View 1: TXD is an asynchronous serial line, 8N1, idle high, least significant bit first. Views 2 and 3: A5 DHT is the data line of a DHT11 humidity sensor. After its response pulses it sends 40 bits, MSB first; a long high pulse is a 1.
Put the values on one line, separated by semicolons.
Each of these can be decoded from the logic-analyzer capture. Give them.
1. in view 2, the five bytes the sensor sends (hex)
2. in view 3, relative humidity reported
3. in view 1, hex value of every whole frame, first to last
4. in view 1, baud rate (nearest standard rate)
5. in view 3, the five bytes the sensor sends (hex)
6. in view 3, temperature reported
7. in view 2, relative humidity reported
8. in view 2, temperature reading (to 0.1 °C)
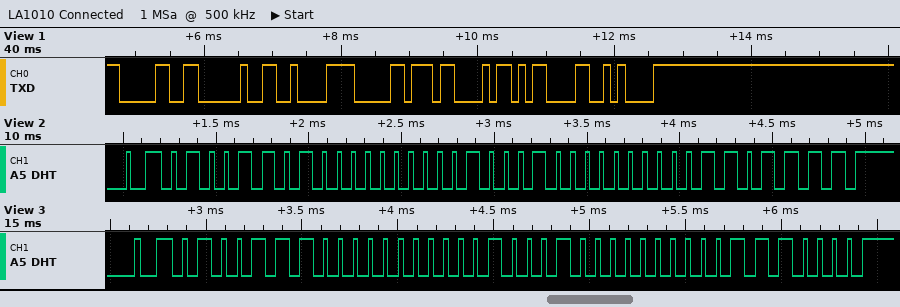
4D 00 22 00 6F; 78 %; 0x30 0x20 0xC2 0xB0 0x43 0x0D 0x0A; 9600 baud; 4E 00 22 00 70; 34.0 °C; 77 %; 34.0 °C
